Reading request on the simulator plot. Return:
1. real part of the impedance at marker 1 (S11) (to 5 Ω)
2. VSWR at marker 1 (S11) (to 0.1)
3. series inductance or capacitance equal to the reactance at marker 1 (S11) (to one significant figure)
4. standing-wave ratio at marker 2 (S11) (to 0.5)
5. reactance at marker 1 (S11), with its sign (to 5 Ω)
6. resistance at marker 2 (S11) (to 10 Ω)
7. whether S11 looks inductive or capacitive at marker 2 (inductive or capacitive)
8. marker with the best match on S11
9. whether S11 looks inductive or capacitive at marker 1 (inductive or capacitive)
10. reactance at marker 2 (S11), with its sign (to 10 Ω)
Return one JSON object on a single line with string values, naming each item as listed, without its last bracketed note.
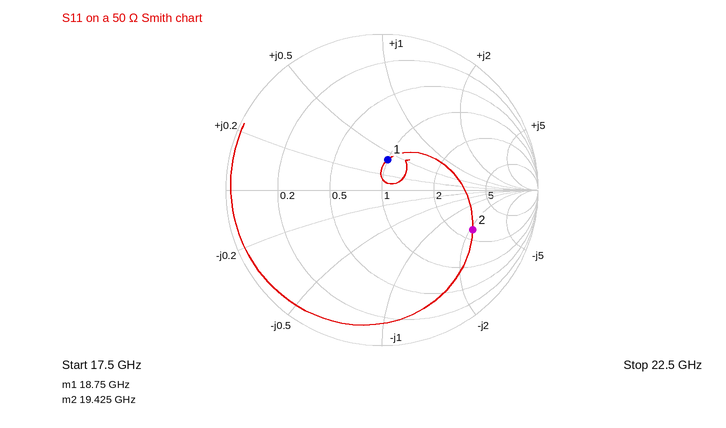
{"real part of the impedance at marker 1 (S11)": "50 Ω", "VSWR at marker 1 (S11)": "1.5", "series inductance or capacitance equal to the reactance at marker 1 (S11)": "200 pH", "standing-wave ratio at marker 2 (S11)": "4.5", "reactance at marker 1 (S11), with its sign": "+20 Ω", "resistance at marker 2 (S11)": "120 Ω", "whether S11 looks inductive or capacitive at marker 2": "capacitive", "marker with the best match on S11": "marker 1", "whether S11 looks inductive or capacitive at marker 1": "inductive", "reactance at marker 2 (S11), with its sign": "-110 Ω"}
